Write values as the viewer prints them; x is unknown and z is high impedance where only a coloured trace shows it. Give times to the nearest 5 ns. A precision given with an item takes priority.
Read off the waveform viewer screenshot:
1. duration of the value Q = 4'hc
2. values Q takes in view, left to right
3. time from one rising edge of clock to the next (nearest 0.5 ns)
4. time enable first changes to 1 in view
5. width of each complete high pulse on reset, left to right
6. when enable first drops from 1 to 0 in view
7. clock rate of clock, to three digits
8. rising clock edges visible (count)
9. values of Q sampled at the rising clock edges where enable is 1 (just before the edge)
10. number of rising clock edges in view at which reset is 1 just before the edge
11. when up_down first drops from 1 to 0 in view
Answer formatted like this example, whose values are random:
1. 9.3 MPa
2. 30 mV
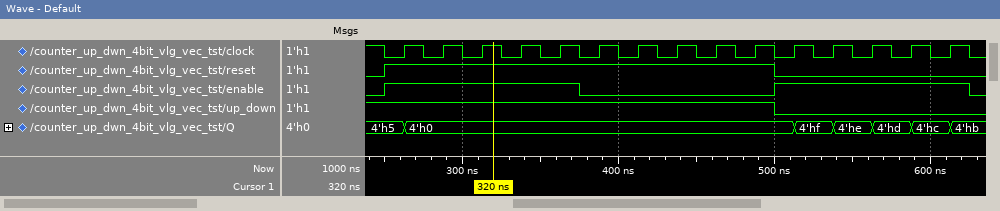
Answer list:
1. 25 ns
2. 4'h5, 4'h0, 4'hf, 4'he, 4'hd, 4'hc, 4'hb
3. 25 ns
4. 250 ns
5. 250 ns
6. 375 ns
7. 40.0 MHz
8. 15
9. 4'h5, 4'h0, 4'h0, 4'h0, 4'h0, 4'h0, 4'hf, 4'he, 4'hd, 4'hc
10. 10
11. 500 ns
